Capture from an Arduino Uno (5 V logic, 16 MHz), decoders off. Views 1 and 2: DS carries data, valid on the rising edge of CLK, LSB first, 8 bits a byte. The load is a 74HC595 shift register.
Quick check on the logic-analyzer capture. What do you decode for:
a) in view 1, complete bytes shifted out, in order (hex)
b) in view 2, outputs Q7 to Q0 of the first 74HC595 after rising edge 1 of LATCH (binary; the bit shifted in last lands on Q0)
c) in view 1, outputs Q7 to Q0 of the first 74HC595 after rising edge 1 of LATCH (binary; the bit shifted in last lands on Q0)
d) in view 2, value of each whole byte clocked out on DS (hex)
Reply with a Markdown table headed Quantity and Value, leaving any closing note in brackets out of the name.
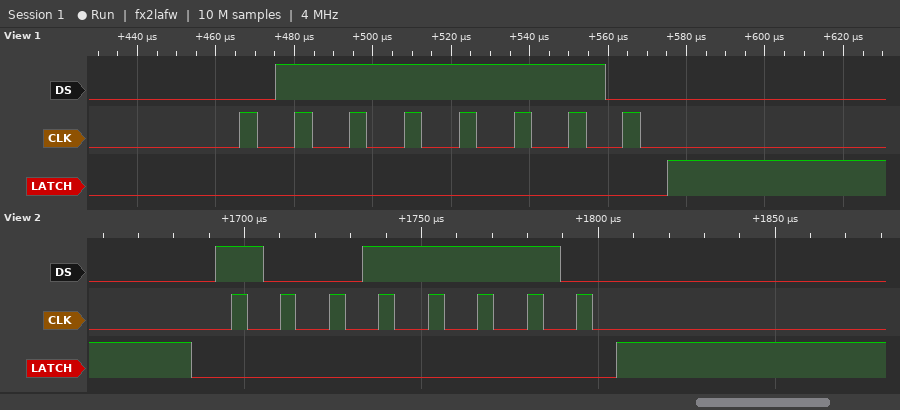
| Quantity | Value |
|---|---|
| in view 1, complete bytes shifted out, in order | 7E |
| in view 2, outputs Q7 to Q0 of the first 74HC595 after rising edge 1 of LATCH | 10011110 |
| in view 1, outputs Q7 to Q0 of the first 74HC595 after rising edge 1 of LATCH | 01111110 |
| in view 2, value of each whole byte clocked out on DS | 0x79 |
